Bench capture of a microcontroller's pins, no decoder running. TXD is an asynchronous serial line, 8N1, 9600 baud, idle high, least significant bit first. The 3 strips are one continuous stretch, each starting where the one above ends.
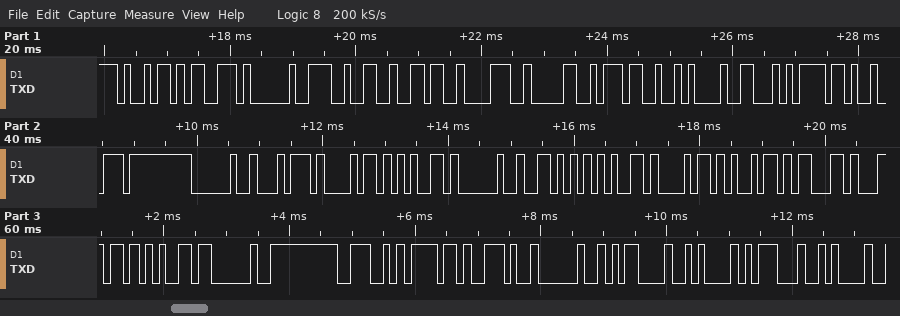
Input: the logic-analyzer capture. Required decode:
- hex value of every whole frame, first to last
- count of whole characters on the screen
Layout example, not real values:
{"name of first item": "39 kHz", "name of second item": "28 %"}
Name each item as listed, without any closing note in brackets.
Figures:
{"hex value of every whole frame, first to last": "69 73 20 32 36 38 30 37 0A 46 6F 72 20 74 68 65 20 56 65 68 69 63 6C 65 20 4E 6F 2E 20 0D 0A 1D 0A", "count of whole characters on the screen": "33"}
